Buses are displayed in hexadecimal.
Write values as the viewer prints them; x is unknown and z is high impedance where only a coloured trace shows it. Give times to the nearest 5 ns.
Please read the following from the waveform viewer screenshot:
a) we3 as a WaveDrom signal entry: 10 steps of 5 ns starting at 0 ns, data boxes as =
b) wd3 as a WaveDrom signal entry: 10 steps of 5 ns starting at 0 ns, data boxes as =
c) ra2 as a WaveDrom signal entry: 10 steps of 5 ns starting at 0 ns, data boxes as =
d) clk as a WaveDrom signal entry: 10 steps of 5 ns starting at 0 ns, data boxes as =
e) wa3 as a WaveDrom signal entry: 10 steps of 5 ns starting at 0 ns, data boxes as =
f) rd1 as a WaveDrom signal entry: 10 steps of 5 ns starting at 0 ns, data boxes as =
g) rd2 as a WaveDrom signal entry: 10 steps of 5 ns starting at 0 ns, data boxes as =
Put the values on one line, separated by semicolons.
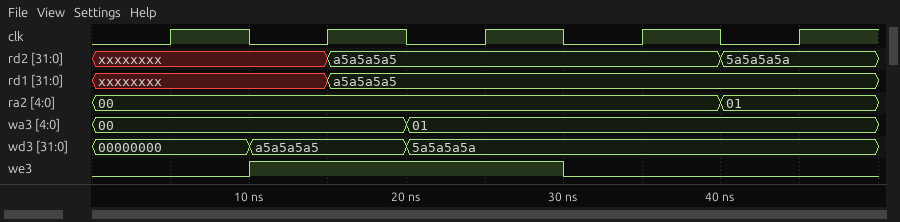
{name: 'we3', wave: '0.1...0...'}; {name: 'wd3', wave: '=.=.=.....', data: '00000000 a5a5a5a5 5a5a5a5a'}; {name: 'ra2', wave: '=.......=.', data: '00 01'}; {name: 'clk', wave: '0101010101'}; {name: 'wa3', wave: '=...=.....', data: '00 01'}; {name: 'rd1', wave: 'x..=......', data: 'a5a5a5a5'}; {name: 'rd2', wave: 'x..=....=.', data: 'a5a5a5a5 5a5a5a5a'}
